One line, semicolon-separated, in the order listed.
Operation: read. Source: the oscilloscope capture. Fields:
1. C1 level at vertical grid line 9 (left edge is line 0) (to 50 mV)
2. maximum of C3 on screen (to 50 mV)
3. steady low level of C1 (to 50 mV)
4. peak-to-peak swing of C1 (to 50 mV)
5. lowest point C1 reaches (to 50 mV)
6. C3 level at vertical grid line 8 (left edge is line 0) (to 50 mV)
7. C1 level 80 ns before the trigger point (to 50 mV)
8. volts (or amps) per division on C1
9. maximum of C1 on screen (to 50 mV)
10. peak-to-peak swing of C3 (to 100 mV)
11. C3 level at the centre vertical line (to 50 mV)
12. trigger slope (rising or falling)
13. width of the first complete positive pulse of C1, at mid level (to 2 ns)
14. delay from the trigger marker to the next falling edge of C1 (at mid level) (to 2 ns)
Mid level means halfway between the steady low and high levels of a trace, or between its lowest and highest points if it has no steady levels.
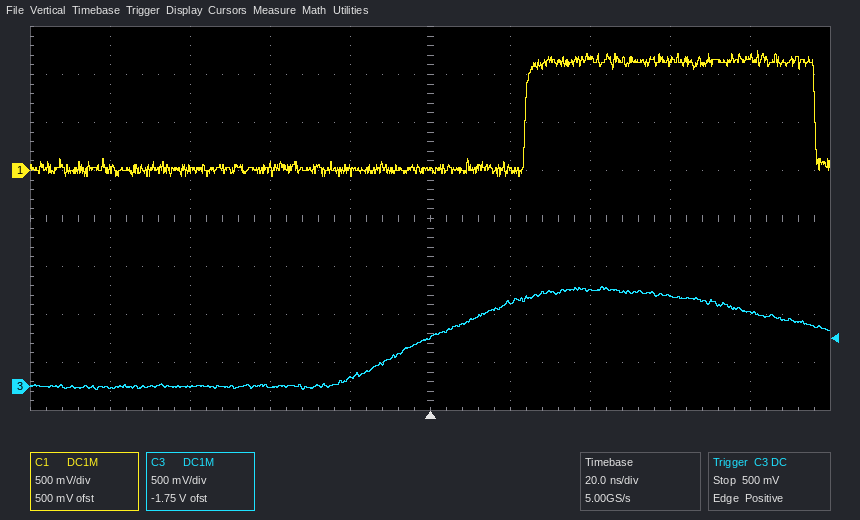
1.15 V; 1.05 V; 0 mV; 1.30 V; -50 mV; 950 mV; 0 mV; 500 mV; 1.25 V; 1.10 V; 500 mV; rising; 72 ns; 96 ns
